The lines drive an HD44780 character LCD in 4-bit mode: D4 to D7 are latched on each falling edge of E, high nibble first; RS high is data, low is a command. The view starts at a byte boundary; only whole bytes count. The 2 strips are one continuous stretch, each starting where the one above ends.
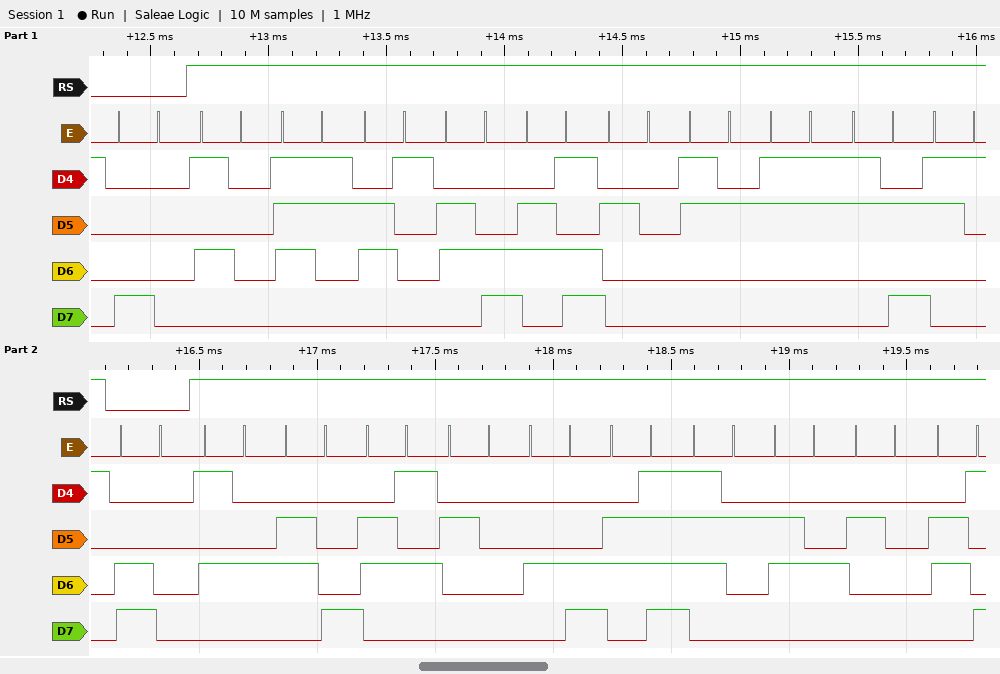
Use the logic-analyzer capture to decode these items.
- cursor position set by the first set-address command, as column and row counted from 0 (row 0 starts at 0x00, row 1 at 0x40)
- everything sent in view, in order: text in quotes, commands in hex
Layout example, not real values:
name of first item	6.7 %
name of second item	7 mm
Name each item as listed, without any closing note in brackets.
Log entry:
cursor position set by the first set-address command, as column and row counted from 0	column 0, row 0
everything sent in view, in order: text in quotes, commands in hex	0x80 "Psalm 23:1" 0xC0 "The Lord i"
